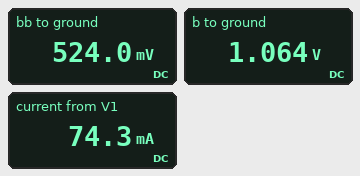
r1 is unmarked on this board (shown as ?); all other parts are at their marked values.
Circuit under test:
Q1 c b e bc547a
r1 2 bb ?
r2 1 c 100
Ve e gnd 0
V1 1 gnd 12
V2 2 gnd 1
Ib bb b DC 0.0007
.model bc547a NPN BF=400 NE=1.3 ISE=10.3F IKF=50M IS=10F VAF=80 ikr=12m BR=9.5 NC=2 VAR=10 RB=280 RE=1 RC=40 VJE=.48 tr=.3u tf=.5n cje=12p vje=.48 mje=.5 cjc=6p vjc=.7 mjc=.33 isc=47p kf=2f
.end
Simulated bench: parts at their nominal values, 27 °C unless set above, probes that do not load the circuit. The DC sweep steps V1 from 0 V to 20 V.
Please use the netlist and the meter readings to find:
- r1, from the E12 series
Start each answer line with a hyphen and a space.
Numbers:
- 680 Ω
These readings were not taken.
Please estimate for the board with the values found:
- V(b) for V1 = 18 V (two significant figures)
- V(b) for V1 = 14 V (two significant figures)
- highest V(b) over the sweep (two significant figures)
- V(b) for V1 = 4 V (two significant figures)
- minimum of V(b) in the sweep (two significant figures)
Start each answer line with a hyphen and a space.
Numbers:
- 1.1 V
- 1.1 V
- 1.1 V
- 990 mV
- 900 mV
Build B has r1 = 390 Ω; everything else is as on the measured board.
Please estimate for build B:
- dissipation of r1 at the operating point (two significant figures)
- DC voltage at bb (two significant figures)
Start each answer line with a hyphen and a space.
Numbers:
- 190 µW
- 730 mV
